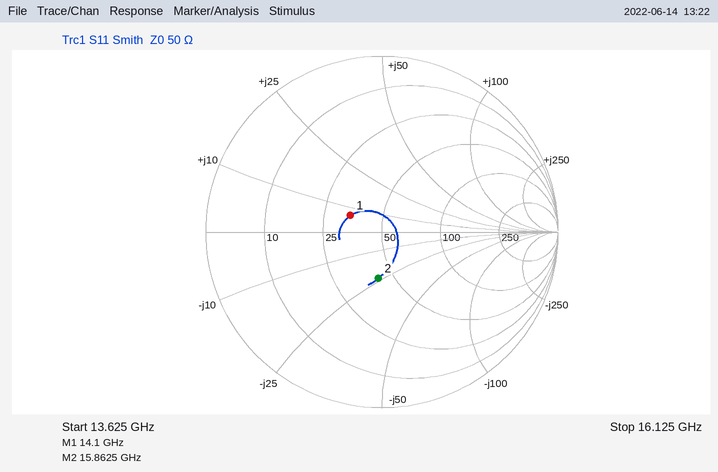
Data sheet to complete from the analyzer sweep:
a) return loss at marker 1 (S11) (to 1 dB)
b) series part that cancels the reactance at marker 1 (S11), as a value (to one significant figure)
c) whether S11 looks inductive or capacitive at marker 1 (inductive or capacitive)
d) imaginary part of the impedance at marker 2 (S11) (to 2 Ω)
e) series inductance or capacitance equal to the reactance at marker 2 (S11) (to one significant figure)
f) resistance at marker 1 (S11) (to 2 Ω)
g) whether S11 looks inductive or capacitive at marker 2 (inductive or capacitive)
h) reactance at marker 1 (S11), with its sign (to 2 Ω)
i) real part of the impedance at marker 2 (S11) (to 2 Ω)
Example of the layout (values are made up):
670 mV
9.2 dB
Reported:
14 dB
2 pF
inductive
-24 Ω
400 fF
34 Ω
capacitive
+6 Ω
42 Ω
